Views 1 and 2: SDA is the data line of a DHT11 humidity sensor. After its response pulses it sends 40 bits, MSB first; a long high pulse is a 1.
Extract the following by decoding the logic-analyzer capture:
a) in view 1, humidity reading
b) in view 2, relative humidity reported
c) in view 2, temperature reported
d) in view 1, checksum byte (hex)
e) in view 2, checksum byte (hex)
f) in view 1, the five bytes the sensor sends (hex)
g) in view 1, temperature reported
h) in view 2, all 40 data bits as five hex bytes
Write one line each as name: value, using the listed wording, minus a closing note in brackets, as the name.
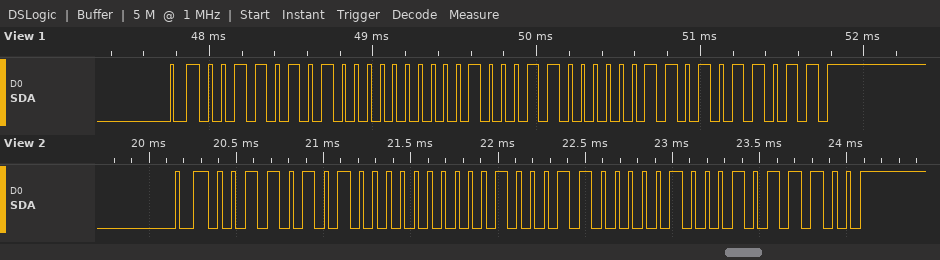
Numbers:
in view 1, humidity reading: 53 %
in view 2, relative humidity reported: 53 %
in view 2, temperature reported: 35.4 °C
in view 1, checksum byte: 0x5B
in view 2, checksum byte: 0x5C
in view 1, the five bytes the sensor sends: 35 00 23 03 5B
in view 1, temperature reported: 35.3 °C
in view 2, all 40 data bits as five hex bytes: 35 00 23 04 5C
